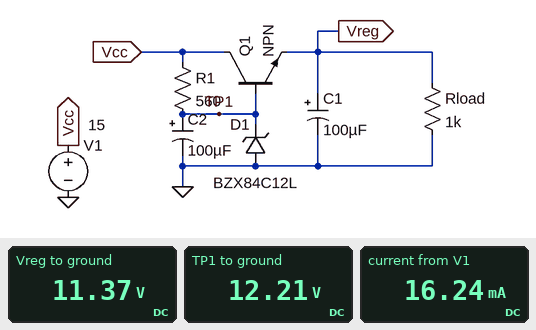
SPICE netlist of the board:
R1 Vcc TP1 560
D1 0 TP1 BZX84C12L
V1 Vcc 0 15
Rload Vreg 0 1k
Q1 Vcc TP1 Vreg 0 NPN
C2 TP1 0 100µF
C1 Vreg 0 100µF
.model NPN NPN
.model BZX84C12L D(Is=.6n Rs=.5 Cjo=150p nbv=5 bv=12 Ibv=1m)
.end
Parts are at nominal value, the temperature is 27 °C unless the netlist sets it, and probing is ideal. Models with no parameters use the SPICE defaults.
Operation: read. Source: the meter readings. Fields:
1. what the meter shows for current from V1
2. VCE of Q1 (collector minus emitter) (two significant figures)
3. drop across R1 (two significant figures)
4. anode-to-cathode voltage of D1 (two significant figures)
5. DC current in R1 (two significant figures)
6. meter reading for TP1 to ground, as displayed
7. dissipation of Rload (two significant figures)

16.24 mA
3.6 V
2.8 V
-12 V
5.0 mA
12.21 V
130 mW
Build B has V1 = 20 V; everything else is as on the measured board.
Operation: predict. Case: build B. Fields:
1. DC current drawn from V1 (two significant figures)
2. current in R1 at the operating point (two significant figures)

25 mA
14 mA
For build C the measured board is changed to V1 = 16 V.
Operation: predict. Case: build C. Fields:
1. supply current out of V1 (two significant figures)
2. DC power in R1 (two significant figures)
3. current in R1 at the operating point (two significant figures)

18 mA
25 mW
6.7 mA
